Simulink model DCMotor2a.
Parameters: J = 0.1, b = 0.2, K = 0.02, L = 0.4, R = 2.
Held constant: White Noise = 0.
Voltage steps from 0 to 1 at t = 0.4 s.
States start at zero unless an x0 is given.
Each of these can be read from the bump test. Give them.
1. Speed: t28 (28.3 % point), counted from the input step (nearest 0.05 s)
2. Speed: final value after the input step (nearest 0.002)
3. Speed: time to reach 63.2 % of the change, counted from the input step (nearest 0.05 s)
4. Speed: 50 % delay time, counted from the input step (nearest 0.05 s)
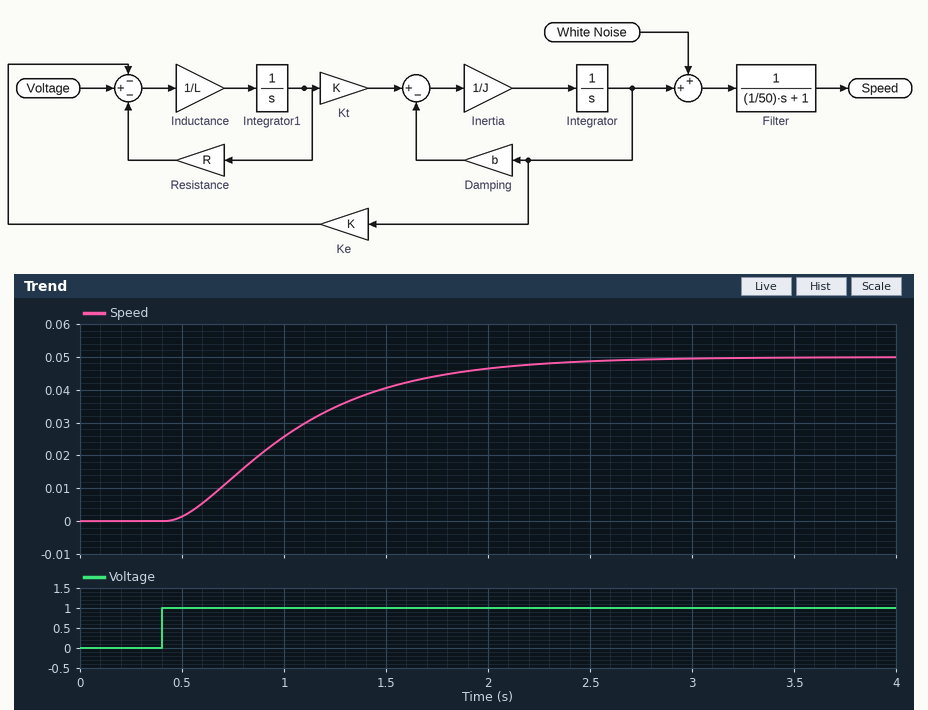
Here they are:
0.35 s
0.050
0.75 s
0.60 s
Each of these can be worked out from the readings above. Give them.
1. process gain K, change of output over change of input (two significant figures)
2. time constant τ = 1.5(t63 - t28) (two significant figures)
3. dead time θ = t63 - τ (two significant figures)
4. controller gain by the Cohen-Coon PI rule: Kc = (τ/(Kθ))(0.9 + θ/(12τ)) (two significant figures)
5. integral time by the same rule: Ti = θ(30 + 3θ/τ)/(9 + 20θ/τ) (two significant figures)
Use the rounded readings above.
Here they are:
0.050
0.60 s
0.15 s
74
0.33 s
